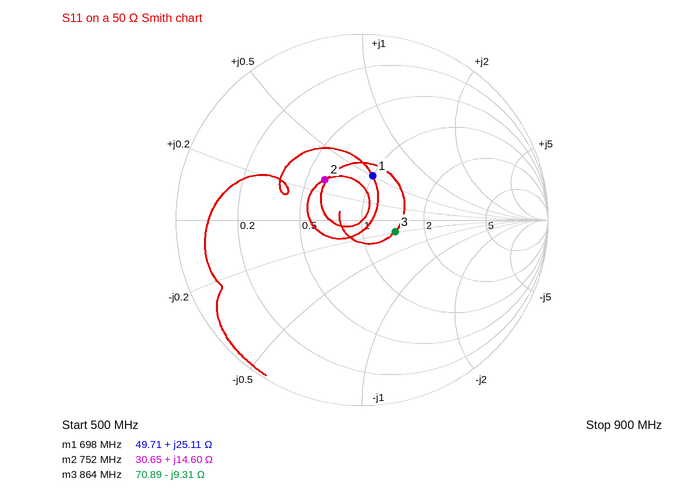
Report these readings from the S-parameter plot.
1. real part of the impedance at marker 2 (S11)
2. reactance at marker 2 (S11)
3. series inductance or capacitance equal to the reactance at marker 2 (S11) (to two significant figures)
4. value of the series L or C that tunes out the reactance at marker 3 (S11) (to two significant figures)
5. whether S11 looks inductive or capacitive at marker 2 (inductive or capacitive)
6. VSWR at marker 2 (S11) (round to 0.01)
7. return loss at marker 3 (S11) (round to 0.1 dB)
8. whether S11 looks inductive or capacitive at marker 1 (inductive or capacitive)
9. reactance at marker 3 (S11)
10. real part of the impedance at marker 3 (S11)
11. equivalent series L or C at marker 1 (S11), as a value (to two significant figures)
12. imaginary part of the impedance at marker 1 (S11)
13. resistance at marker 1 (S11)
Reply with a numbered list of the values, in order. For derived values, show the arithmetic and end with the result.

1. 30.65 Ω
2. +14.60 Ω
3. L = 14.6 Ω/(2π × 752 MHz) ≈ 3.1 nH
4. L = 9.31 Ω/(2π × 864 MHz) ≈ 1.7 nH
5. inductive
6. 1.84
7. 14.5 dB
8. inductive
9. -9.31 Ω
10. 70.89 Ω
11. L = 25.11 Ω/(2π × 698 MHz) ≈ 5.7 nH
12. +25.11 Ω
13. 49.71 Ω
